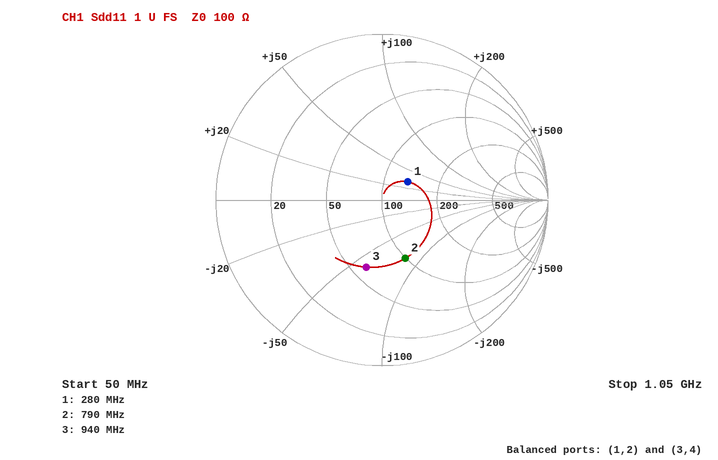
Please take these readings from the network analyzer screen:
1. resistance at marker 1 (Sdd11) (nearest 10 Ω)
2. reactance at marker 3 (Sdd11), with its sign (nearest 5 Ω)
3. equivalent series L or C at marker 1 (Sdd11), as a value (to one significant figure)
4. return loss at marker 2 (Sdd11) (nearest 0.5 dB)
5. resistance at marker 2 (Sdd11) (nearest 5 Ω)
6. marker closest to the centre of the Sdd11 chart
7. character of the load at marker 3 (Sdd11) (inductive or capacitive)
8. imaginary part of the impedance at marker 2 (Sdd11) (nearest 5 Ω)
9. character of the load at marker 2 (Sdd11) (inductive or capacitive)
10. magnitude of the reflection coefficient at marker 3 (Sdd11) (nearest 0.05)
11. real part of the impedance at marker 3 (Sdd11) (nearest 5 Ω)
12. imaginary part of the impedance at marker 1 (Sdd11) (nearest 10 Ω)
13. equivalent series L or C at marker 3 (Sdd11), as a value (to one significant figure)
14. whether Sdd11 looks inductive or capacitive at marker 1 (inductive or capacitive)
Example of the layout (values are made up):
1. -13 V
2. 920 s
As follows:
1. 130 Ω
2. -60 Ω
3. 20 nH
4. 8.5 dB
5. 100 Ω
6. marker 1
7. capacitive
8. -80 Ω
9. capacitive
10. 0.40
11. 60 Ω
12. +30 Ω
13. 3 pF
14. inductive
